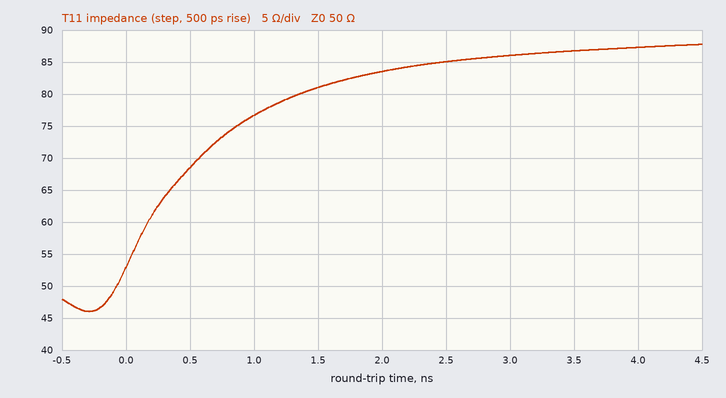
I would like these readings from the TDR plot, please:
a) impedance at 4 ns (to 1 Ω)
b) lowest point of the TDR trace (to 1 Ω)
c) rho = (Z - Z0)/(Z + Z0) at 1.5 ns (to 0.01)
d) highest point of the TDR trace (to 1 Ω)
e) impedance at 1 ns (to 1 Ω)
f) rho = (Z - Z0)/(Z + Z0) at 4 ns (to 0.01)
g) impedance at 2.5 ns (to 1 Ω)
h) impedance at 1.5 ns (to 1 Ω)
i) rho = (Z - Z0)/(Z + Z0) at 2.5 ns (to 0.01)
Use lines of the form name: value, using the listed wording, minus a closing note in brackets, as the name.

impedance at 4 ns: 87 Ω
lowest point of the TDR trace: 46 Ω
rho = (Z - Z0)/(Z + Z0) at 1.5 ns: +0.24
highest point of the TDR trace: 88 Ω
impedance at 1 ns: 77 Ω
rho = (Z - Z0)/(Z + Z0) at 4 ns: +0.27
impedance at 2.5 ns: 85 Ω
impedance at 1.5 ns: 81 Ω
rho = (Z - Z0)/(Z + Z0) at 2.5 ns: +0.26
